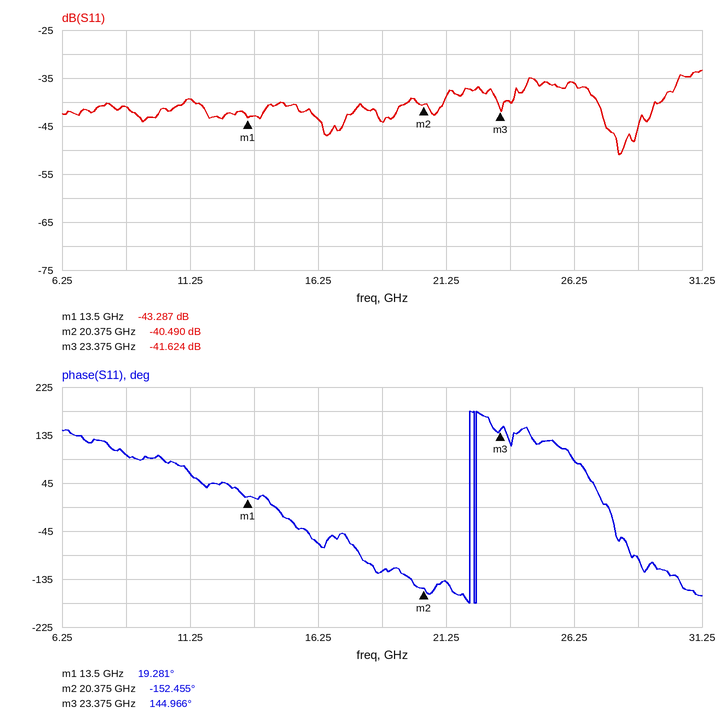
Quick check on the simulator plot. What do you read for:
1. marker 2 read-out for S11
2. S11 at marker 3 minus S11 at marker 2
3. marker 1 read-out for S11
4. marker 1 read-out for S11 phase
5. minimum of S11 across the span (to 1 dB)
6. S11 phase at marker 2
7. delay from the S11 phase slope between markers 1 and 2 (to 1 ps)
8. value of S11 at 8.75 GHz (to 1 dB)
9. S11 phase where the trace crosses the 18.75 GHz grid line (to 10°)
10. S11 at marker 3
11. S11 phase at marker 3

-40.490 dB
-1.134 dB
-43.287 dB
19.281°
-51 dB
-152.455°
69 ps
-41 dB
-120°
-41.624 dB
144.966°
